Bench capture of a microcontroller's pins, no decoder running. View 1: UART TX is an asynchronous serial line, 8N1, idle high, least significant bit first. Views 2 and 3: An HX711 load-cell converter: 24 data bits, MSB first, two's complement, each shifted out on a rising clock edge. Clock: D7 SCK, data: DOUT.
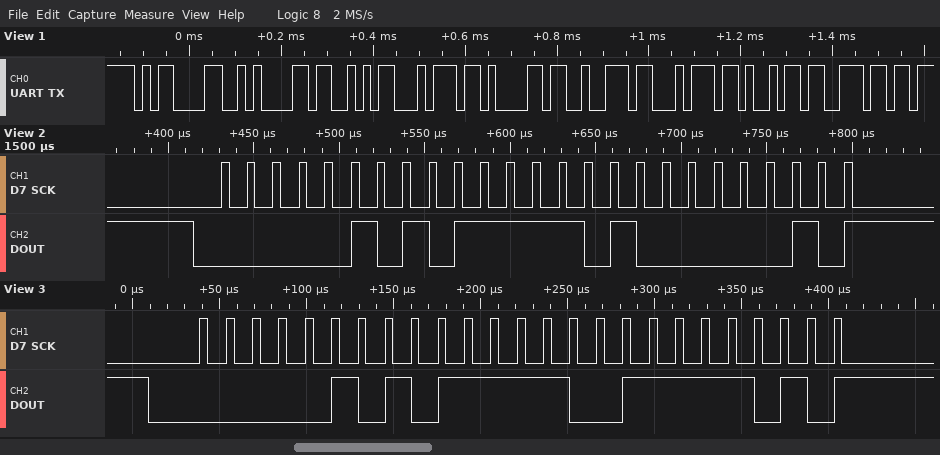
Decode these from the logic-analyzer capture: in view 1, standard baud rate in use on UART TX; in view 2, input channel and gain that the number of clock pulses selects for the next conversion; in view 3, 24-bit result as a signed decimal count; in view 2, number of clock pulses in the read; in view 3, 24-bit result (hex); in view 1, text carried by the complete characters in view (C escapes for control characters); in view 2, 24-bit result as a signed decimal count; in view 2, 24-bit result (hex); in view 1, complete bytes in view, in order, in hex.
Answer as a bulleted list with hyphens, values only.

- 57600 baud
- channel A, gain 128
- 359674
- 25
- 0x057CFA
- "\r\nStartin"
- 359682
- 0x057D02
- 0D 0A 53 74 61 72 74 69 6E
